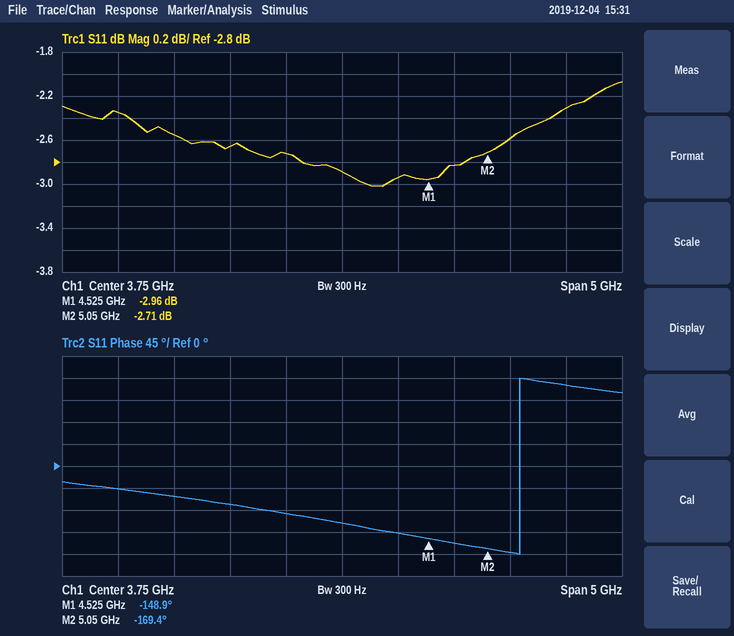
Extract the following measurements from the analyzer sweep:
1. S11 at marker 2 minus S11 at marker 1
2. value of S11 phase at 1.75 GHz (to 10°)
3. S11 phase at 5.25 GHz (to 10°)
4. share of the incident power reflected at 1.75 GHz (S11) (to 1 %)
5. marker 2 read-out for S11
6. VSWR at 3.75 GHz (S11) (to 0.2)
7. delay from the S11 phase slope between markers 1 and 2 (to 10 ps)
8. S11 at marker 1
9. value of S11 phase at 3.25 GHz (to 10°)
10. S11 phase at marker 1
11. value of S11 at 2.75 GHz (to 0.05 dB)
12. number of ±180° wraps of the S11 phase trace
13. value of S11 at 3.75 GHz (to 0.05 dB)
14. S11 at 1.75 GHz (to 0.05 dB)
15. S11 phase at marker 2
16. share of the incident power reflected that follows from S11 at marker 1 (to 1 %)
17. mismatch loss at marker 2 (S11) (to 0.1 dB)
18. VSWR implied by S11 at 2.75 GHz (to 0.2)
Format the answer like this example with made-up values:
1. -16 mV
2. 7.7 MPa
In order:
1. 0.25 dB
2. -50°
3. -180°
4. 58 %
5. -2.71 dB
6. 6.0
7. 110 ps
8. -2.96 dB
9. -100°
10. -148.9°
11. -2.65 dB
12. 1
13. -2.90 dB
14. -2.35 dB
15. -169.4°
16. 51 %
17. 3.3 dB
18. 6.6
